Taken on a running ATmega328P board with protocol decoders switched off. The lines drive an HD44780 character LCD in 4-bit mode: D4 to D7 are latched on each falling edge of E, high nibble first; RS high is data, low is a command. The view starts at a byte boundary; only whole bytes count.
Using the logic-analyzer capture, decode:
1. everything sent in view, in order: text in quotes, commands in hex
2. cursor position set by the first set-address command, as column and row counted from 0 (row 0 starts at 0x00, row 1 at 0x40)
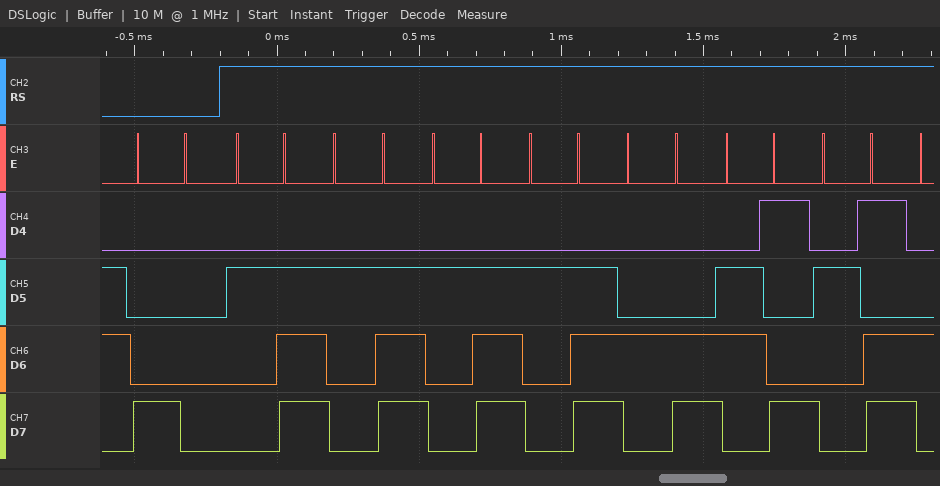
0x80 "....Li-"
column 0, row 0
